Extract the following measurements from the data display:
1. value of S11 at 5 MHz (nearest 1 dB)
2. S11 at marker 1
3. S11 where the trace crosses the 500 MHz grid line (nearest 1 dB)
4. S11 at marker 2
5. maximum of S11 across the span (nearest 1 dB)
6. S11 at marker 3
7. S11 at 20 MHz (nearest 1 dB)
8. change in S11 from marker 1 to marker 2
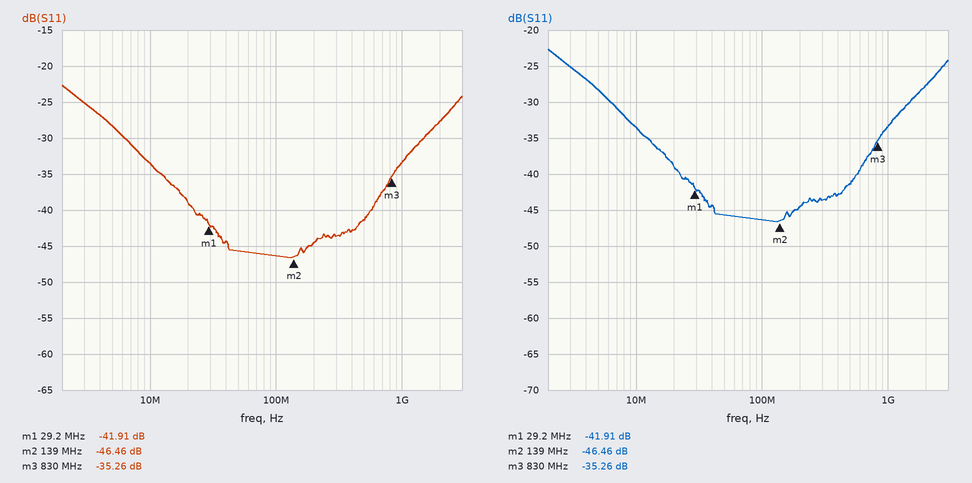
-28 dB
-41.91 dB
-41 dB
-46.46 dB
-23 dB
-35.26 dB
-39 dB
-4.55 dB
